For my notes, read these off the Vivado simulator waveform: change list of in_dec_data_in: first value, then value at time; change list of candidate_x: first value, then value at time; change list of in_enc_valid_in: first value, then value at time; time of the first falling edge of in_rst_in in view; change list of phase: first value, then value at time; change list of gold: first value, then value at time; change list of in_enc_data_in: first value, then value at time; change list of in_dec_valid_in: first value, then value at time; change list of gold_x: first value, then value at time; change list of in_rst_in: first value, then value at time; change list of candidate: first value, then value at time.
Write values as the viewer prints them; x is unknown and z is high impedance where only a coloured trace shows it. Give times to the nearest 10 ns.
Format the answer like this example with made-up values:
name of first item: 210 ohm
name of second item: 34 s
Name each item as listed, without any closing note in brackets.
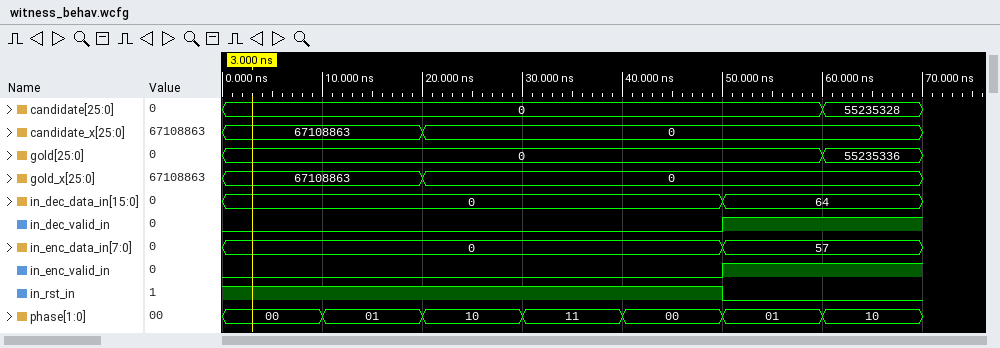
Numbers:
change list of in_dec_data_in: first value, then value at time: 0, 64 at 50 ns
change list of candidate_x: first value, then value at time: 67108863, 0 at 20 ns
change list of in_enc_valid_in: first value, then value at time: 0, 1 at 50 ns
time of the first falling edge of in_rst_in in view: 50 ns
change list of phase: first value, then value at time: 00, 01 at 10 ns, 10 at 20 ns, 11 at 30 ns, 00 at 40 ns, 01 at 50 ns, 10 at 60 ns
change list of gold: first value, then value at time: 0, 55235336 at 60 ns
change list of in_enc_data_in: first value, then value at time: 0, 57 at 50 ns
change list of in_dec_valid_in: first value, then value at time: 0, 1 at 50 ns
change list of gold_x: first value, then value at time: 67108863, 0 at 20 ns
change list of in_rst_in: first value, then value at time: 1, 0 at 50 ns
change list of candidate: first value, then value at time: 0, 55235328 at 60 ns
